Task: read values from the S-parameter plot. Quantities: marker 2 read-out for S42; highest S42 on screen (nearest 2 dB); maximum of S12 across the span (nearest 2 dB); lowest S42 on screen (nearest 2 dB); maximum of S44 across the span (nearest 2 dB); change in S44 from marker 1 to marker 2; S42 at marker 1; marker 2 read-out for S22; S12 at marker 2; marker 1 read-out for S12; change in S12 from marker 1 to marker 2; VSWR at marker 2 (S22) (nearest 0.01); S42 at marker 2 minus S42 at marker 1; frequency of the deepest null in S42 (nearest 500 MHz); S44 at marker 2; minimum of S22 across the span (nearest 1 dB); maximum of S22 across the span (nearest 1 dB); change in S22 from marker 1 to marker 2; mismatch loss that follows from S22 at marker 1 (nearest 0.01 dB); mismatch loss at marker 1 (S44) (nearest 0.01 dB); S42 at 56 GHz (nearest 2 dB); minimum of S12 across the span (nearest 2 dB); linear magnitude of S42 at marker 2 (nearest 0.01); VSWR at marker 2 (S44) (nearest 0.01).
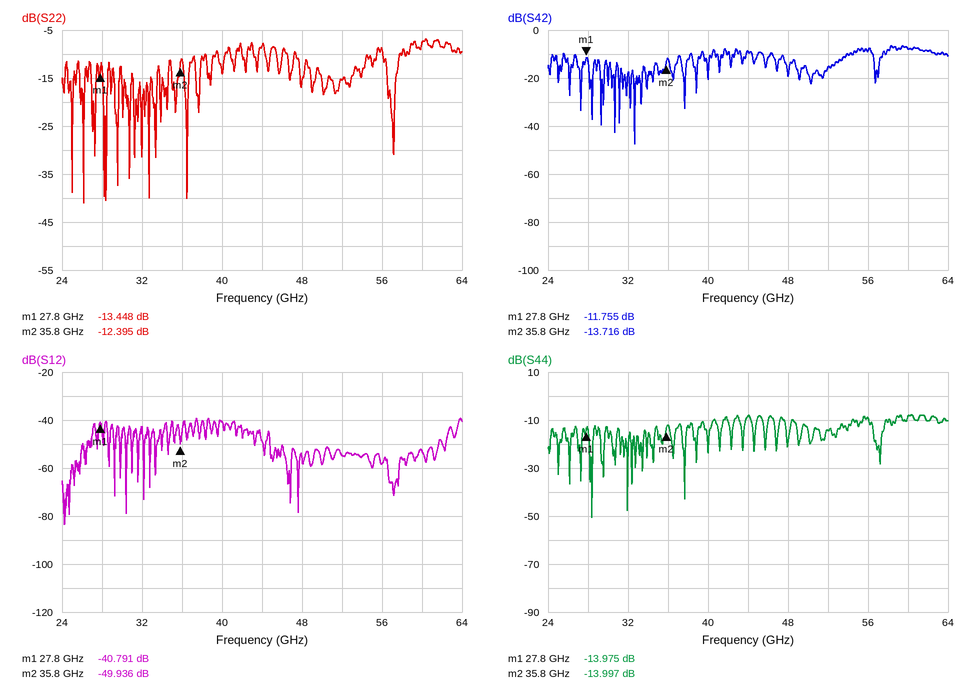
-13.716 dB
-6 dB
-40 dB
-48 dB
-8 dB
-0.022 dB
-11.755 dB
-12.395 dB
-49.936 dB
-40.791 dB
-9.145 dB
1.63
-1.961 dB
32.5 GHz
-13.997 dB
-41 dB
-7 dB
1.053 dB
0.20 dB
0.18 dB
-8 dB
-84 dB
0.21
1.50
